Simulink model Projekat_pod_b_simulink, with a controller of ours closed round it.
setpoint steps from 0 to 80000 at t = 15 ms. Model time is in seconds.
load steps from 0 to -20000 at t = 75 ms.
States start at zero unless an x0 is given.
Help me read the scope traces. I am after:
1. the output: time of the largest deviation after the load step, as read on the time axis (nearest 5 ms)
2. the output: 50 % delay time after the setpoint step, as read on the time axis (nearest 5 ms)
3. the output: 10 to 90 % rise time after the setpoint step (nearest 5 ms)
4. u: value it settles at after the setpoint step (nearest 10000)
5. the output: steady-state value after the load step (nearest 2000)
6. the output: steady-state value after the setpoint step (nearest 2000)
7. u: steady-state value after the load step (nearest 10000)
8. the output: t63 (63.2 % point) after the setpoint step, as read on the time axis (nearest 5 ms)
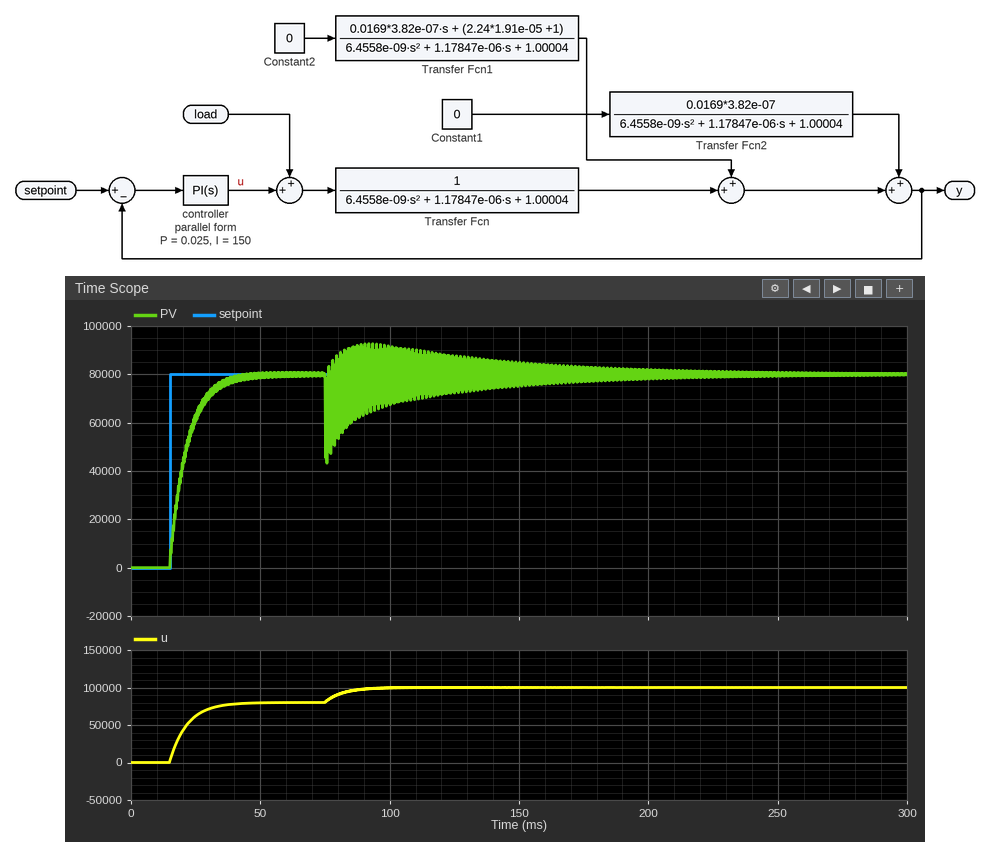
75 ms
20 ms
15 ms
80000
80000
80000
100000
20 ms
